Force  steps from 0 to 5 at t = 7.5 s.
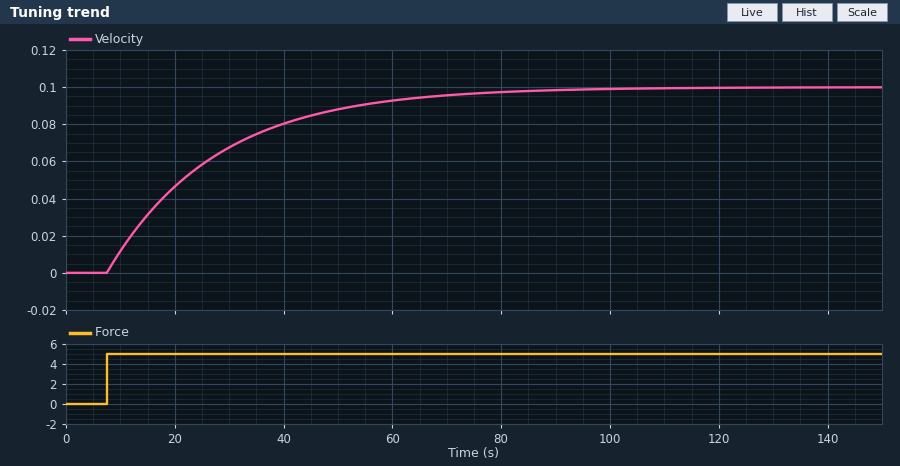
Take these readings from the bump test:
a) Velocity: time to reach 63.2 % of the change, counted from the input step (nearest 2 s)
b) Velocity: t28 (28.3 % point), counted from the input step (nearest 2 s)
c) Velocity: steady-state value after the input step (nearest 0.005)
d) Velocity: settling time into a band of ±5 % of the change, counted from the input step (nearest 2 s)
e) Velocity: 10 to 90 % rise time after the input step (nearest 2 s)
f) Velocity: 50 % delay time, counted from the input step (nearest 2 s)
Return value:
20 s
6 s
0.100
60 s
44 s
14 s
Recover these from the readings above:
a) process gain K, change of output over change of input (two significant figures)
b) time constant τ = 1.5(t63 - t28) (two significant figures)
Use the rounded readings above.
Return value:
0.020
21 s
